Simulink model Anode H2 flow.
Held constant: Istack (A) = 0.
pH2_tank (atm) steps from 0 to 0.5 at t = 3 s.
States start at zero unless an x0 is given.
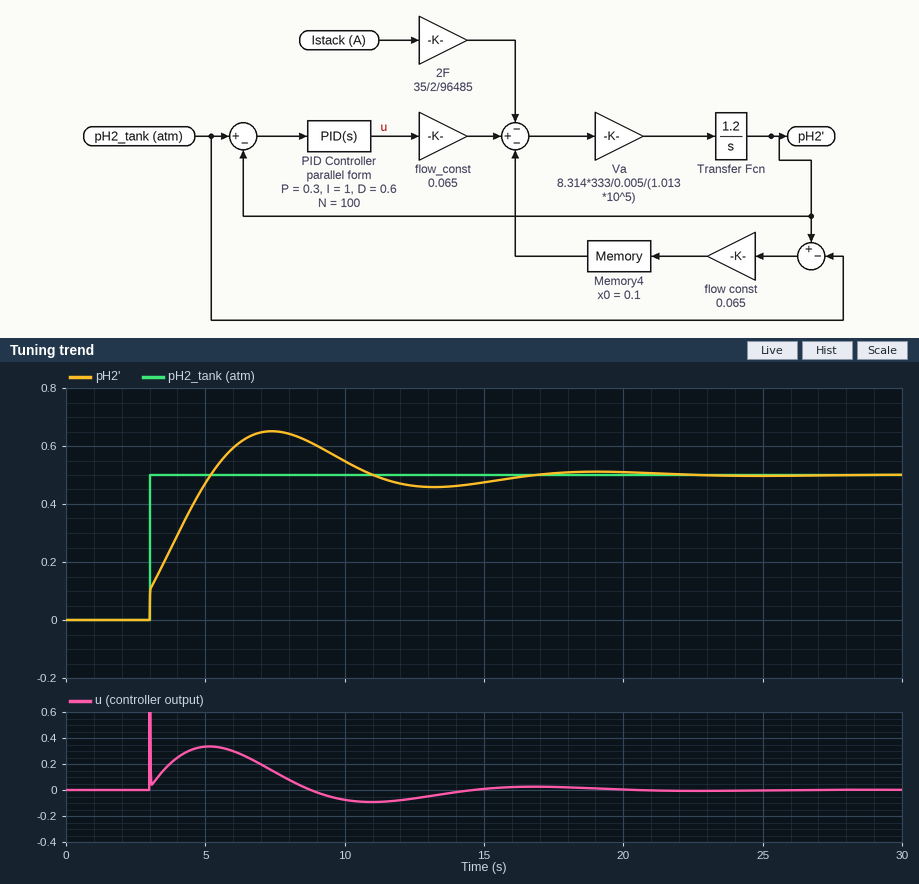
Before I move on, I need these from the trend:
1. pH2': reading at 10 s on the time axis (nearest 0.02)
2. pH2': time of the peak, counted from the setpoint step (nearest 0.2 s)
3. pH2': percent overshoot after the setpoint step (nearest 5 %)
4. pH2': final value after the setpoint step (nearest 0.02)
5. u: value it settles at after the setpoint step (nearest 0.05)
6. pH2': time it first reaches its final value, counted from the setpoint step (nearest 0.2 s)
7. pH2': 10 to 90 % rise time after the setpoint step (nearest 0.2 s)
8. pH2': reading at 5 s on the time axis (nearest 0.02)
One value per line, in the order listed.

0.54
4.4 s
30 %
0.50
0.00
2.2 s
1.8 s
0.48
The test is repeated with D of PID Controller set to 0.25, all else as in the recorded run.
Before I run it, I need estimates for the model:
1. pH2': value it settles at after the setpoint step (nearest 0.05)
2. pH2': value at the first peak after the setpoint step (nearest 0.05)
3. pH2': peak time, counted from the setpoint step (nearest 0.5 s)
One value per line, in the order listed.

0.50
0.65
4.0 s
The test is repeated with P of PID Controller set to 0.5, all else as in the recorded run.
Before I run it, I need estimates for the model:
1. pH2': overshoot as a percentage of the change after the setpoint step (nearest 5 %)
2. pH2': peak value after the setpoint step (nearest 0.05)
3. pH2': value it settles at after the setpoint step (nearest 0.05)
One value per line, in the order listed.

25 %
0.65
0.50
